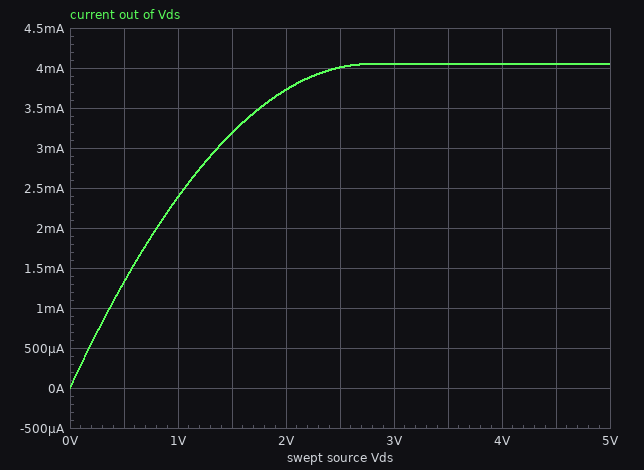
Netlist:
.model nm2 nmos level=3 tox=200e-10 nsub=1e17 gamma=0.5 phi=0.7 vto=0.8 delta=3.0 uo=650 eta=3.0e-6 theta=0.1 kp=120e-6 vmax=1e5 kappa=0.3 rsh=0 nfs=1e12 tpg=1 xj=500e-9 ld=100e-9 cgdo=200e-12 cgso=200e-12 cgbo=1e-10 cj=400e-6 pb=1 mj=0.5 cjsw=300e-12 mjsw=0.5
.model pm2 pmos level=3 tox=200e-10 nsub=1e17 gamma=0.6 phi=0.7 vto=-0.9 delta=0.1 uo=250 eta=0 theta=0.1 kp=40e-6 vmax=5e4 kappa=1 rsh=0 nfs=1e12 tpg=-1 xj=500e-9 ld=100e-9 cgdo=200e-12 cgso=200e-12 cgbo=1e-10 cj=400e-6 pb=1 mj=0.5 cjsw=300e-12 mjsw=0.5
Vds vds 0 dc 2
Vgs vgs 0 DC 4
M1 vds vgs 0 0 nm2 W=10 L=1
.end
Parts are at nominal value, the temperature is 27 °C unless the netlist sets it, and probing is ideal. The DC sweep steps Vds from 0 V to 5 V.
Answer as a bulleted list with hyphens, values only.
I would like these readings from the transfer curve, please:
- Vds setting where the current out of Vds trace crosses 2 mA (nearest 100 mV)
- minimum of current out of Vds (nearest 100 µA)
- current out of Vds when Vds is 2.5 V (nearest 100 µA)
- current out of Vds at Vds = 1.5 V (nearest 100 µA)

- 800 mV
- 0 A
- 4.0 mA
- 3.2 mA
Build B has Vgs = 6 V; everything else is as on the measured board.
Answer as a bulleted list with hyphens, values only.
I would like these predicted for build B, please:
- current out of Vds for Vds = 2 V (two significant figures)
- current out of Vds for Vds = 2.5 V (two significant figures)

- 6.4 mA
- 7.4 mA
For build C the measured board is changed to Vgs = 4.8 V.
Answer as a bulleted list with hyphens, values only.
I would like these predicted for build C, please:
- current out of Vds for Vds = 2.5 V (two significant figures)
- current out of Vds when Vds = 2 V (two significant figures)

- 5.5 mA
- 4.9 mA
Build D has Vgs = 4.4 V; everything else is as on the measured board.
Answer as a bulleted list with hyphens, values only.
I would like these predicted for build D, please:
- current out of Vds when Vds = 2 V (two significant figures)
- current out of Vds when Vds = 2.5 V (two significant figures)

- 4.3 mA
- 4.8 mA
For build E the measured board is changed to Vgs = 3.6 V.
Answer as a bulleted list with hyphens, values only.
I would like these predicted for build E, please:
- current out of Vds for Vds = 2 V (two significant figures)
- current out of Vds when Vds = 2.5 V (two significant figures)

- 3.1 mA
- 3.2 mA
